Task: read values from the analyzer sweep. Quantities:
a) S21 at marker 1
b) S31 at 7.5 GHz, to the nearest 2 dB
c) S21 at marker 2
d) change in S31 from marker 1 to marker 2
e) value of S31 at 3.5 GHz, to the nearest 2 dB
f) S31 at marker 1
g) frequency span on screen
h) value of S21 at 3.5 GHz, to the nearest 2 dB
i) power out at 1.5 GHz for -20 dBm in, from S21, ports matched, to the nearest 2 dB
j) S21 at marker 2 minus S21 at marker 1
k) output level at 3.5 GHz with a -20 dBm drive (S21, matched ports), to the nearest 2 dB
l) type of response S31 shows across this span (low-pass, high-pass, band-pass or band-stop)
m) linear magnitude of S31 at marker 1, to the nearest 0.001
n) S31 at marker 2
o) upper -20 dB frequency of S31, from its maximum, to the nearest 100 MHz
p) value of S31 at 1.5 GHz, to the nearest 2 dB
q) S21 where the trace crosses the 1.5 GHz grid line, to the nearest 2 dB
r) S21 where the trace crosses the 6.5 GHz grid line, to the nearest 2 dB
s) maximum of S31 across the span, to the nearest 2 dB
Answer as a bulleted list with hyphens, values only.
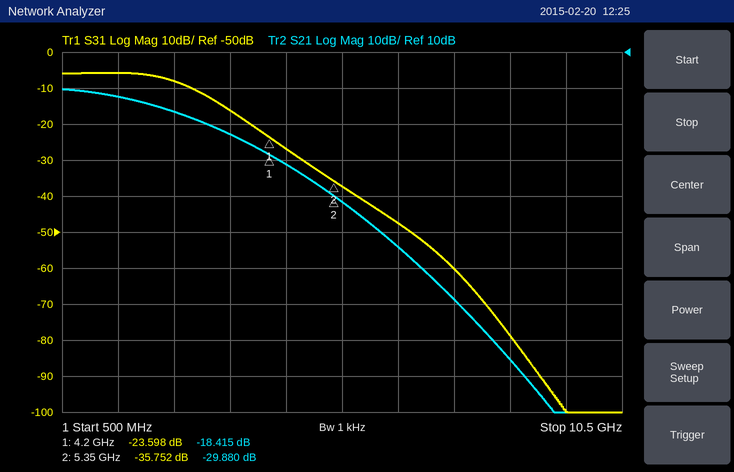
- -18.415 dB
- -60 dB
- -29.880 dB
- -12.154 dB
- -16 dB
- -23.598 dB
- 10 GHz
- -12 dB
- -22 dBm
- -11.465 dB
- -32 dBm
- low-pass
- 0.066
- -35.752 dB
- 4.4 GHz
- -6 dB
- -2 dB
- -44 dB
- -6 dB
